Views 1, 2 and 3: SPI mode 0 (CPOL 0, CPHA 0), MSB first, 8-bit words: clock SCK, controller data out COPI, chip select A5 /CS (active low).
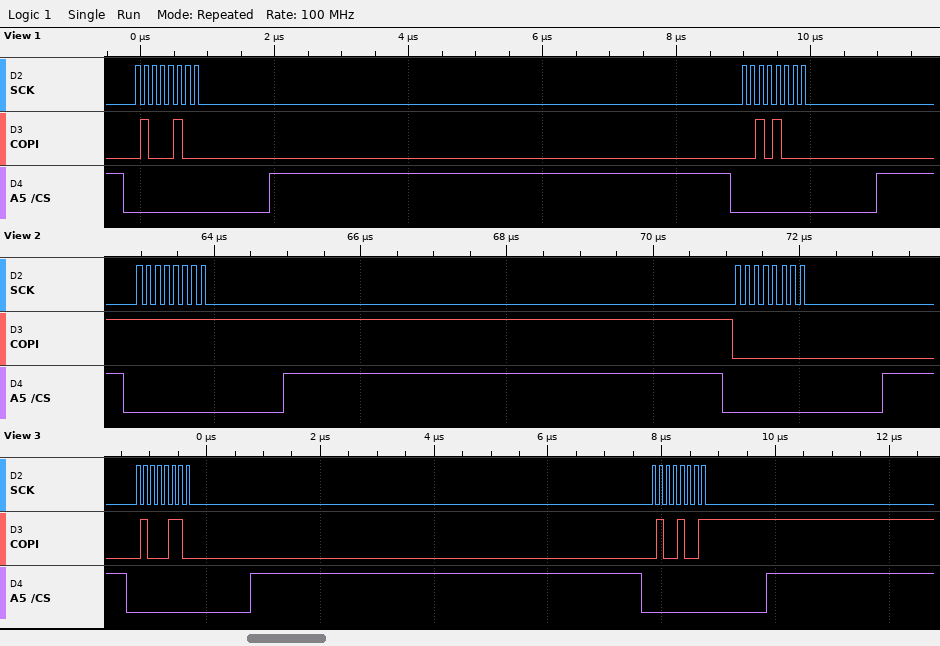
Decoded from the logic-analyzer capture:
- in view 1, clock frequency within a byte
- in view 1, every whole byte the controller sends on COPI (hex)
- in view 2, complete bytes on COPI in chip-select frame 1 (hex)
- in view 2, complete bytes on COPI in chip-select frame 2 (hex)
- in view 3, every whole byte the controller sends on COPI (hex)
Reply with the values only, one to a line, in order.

8 MHz
44 28
FF
00
0x46 0x49
